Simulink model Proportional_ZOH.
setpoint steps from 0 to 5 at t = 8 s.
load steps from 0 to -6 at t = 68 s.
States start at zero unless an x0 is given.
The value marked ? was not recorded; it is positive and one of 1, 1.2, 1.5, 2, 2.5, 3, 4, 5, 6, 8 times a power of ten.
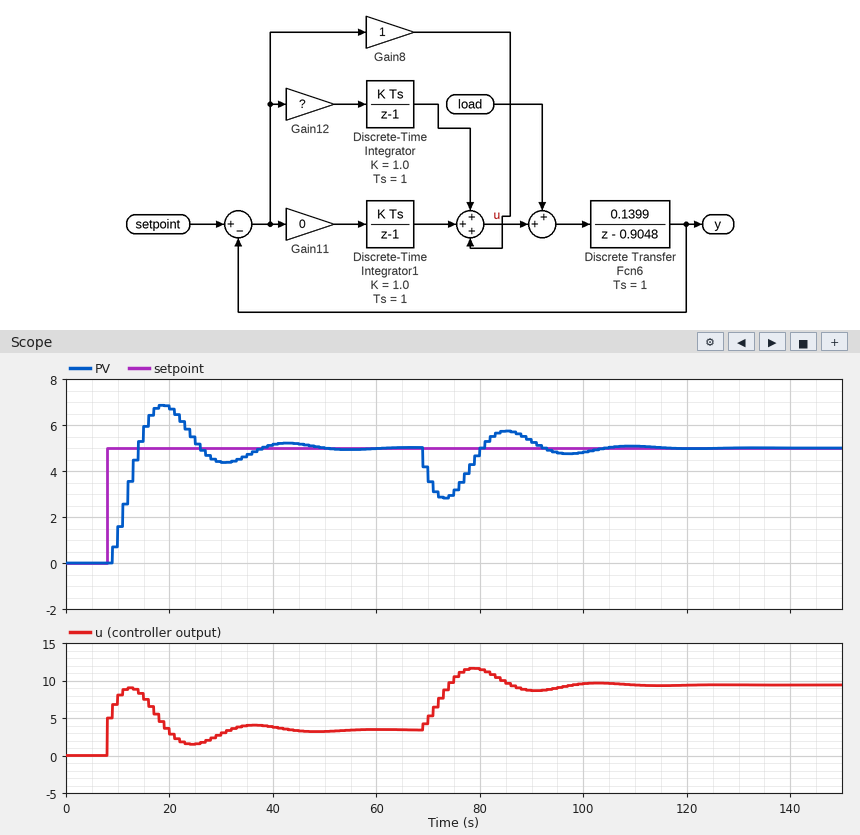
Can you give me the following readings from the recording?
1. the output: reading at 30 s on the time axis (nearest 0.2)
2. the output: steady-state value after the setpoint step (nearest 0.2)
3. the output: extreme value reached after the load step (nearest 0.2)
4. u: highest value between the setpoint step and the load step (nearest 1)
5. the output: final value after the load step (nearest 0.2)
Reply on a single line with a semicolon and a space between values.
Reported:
4.4; 5.0; 2.8; 9; 5.0
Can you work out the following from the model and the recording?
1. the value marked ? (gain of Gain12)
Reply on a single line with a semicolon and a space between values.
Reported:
0.5
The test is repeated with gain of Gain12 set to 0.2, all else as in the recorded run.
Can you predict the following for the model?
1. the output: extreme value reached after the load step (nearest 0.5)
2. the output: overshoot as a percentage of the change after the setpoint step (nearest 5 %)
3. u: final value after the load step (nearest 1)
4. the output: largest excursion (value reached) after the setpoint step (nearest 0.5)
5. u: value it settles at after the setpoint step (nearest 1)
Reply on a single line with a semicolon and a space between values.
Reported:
2.5; 10 %; 9; 5.5; 3
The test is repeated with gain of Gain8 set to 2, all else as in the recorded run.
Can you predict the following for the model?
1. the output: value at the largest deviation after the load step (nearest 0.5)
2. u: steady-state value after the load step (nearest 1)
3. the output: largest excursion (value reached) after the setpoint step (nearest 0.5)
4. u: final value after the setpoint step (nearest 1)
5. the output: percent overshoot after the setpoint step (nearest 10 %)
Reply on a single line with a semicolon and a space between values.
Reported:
3.5; 9; 6.0; 3; 20 %
